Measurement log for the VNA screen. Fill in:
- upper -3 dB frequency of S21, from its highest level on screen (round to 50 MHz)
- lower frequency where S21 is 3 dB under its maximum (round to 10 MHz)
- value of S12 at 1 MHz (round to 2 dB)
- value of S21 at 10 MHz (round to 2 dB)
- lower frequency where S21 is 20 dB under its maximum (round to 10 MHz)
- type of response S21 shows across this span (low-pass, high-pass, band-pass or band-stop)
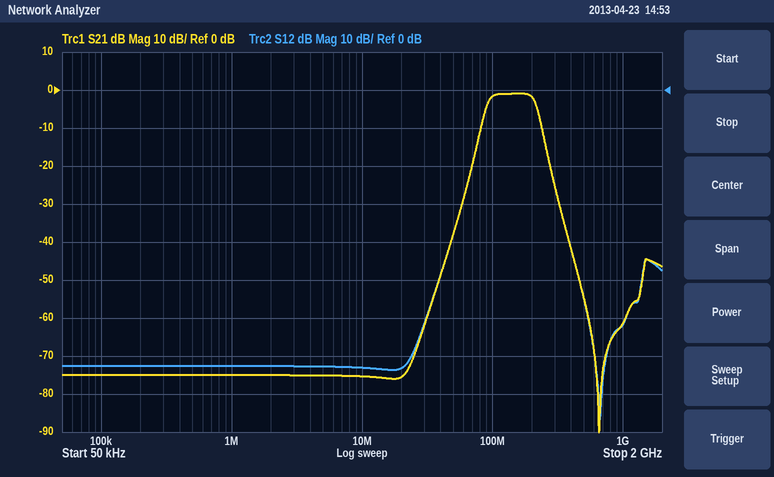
200 MHz
90 MHz
-72 dB
-76 dB
70 MHz
band-pass
